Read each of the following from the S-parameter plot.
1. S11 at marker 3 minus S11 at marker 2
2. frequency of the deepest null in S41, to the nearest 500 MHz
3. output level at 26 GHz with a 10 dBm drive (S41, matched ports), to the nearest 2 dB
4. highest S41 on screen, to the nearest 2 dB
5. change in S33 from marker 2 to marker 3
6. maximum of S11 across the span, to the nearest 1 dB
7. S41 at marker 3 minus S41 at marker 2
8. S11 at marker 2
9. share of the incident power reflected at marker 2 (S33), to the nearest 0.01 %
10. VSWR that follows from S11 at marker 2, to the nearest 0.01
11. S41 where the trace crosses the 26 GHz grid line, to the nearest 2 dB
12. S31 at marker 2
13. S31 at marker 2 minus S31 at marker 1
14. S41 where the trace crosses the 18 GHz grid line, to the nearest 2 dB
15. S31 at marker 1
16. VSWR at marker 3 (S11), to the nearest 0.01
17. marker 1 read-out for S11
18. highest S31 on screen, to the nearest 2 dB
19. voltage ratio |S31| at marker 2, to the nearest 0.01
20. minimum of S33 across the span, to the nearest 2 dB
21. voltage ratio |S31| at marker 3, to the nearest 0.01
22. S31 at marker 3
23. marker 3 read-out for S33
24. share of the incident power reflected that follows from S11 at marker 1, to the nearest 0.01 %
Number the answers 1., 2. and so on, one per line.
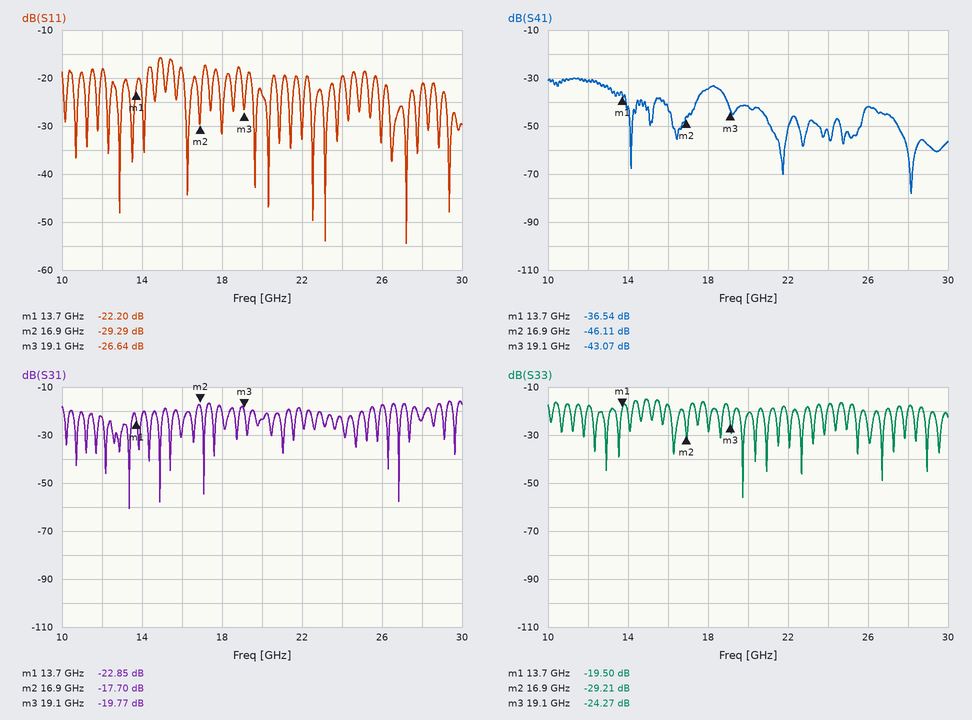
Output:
1. 2.65 dB
2. 28.0 GHz
3. -32 dBm
4. -30 dB
5. 4.94 dB
6. -16 dB
7. 3.04 dB
8. -29.29 dB
9. 0.12 %
10. 1.07
11. -42 dB
12. -17.70 dB
13. 5.15 dB
14. -34 dB
15. -22.85 dB
16. 1.10
17. -22.20 dB
18. -16 dB
19. 0.13
20. -56 dB
21. 0.10
22. -19.77 dB
23. -24.27 dB
24. 0.60 %
